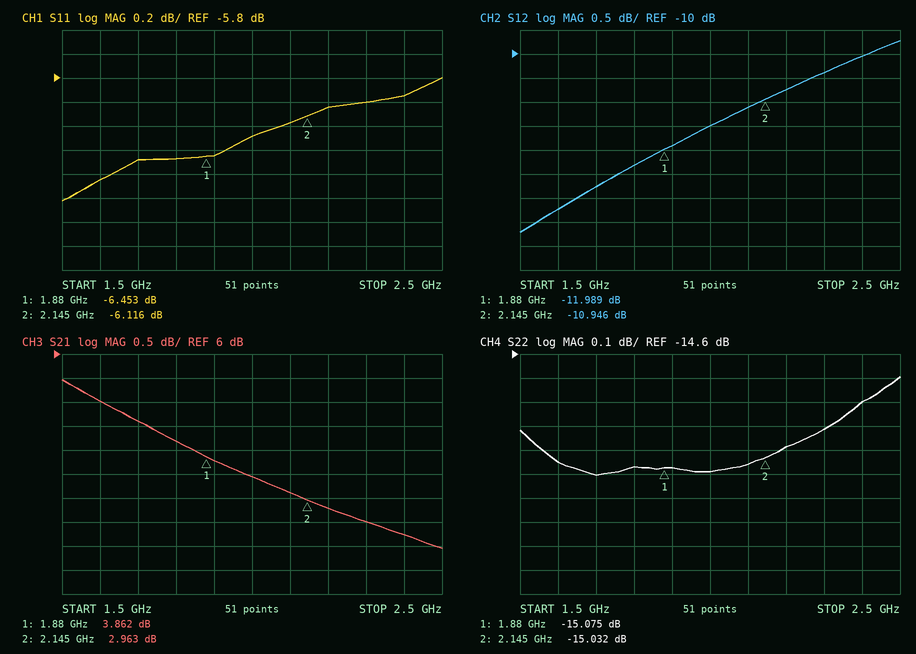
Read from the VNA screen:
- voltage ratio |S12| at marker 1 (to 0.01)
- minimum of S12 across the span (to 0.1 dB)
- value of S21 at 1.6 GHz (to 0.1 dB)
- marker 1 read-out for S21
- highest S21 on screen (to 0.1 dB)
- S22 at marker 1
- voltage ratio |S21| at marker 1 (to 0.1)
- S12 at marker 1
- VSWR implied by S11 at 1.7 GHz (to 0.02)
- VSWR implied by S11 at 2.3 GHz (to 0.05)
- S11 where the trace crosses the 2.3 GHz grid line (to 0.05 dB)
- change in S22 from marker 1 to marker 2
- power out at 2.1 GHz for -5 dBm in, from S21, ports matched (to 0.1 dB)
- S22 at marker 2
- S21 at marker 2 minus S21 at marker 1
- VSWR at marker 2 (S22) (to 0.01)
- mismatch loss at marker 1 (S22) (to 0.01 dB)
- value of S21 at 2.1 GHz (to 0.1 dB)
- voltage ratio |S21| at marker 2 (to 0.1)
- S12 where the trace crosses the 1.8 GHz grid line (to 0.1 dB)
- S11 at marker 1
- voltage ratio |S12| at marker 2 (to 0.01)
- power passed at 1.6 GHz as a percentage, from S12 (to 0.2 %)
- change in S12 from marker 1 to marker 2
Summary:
0.25
-13.7 dB
5.0 dB
3.862 dB
5.5 dB
-15.075 dB
1.6
-11.989 dB
2.80
3.00
-6.00 dB
0.043 dB
-1.9 dBm
-15.032 dB
-0.899 dB
1.43
0.14 dB
3.1 dB
1.4
-12.3 dB
-6.453 dB
0.28
4.8 %
1.043 dB
